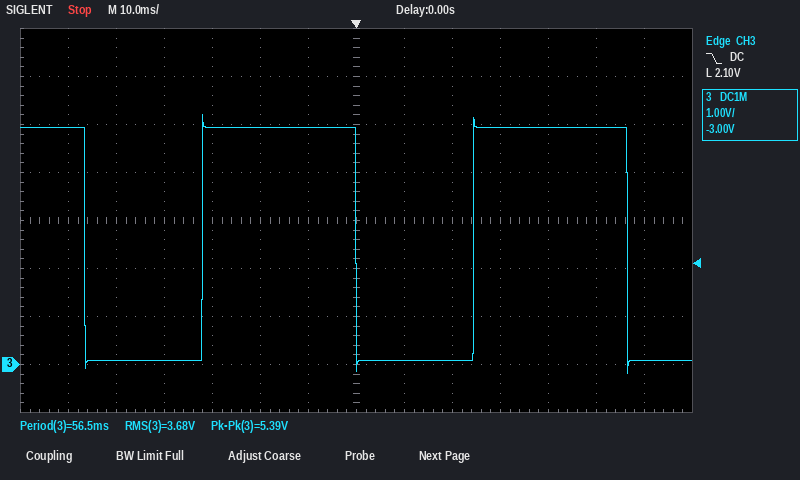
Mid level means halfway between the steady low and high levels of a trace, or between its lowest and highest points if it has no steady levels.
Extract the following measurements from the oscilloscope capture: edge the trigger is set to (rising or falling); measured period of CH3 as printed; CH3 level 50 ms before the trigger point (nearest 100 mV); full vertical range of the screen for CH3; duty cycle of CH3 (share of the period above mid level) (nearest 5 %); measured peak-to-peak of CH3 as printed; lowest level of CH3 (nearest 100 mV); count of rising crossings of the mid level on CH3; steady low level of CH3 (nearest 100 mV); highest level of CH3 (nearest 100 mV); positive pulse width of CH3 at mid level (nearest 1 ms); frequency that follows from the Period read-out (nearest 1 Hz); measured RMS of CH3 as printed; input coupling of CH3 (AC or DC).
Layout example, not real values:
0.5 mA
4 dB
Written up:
falling
56.5 ms
100 mV
8 V
55 %
5.39 V
-200 mV
2
100 mV
5.2 V
32 ms
18 Hz
3.68 V
DC
